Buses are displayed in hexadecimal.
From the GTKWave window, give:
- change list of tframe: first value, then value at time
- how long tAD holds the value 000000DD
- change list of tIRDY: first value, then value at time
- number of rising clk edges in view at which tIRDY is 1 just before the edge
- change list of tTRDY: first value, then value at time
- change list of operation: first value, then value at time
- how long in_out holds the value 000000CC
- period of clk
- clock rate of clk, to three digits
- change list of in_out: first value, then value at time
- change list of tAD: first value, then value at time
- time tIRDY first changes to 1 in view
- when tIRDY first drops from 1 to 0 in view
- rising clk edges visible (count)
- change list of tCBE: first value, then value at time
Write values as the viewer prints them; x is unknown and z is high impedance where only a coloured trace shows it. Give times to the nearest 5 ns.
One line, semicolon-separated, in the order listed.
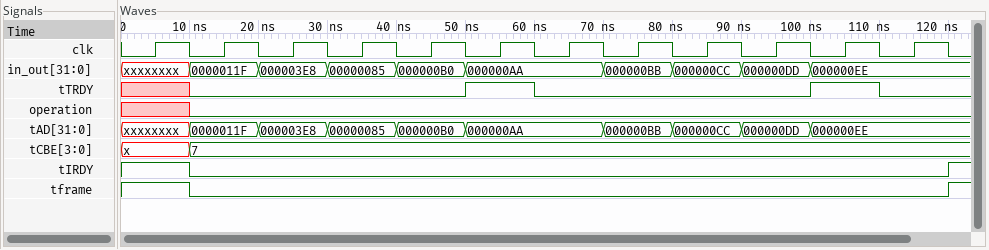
1, 0 at 10 ns, 1 at 120 ns; 10 ns; 1, 0 at 10 ns, 1 at 120 ns; 1; x, 0 at 10 ns, 1 at 50 ns, 0 at 60 ns, 1 at 100 ns, 0 at 110 ns; x, 0 at 10 ns; 10 ns; 10 ns; 100 MHz; xxxxxxxx, 0000011F at 10 ns, 000003E8 at 20 ns, 00000085 at 30 ns, 000000B0 at 40 ns, 000000AA at 50 ns, 000000BB at 70 ns, 000000CC at 80 ns, 000000DD at 90 ns, 000000EE at 100 ns; xxxxxxxx, 0000011F at 10 ns, 000003E8 at 20 ns, 00000085 at 30 ns, 000000B0 at 40 ns, 000000AA at 50 ns, 000000BB at 70 ns, 000000CC at 80 ns, 000000DD at 90 ns, 000000EE at 100 ns; 120 ns; 10 ns; 12; x, 7 at 10 ns
